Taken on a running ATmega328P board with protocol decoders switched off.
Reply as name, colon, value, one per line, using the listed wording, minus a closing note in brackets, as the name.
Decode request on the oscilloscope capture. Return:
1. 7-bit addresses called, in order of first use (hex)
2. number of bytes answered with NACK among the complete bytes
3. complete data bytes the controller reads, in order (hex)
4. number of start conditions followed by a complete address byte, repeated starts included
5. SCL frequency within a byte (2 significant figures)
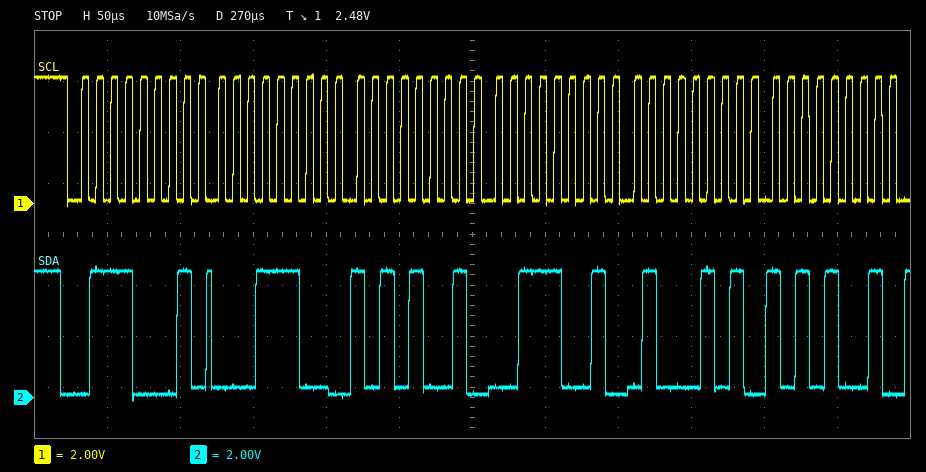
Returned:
7-bit addresses called, in order of first use: 0x38
number of bytes answered with NACK among the complete bytes: 0
complete data bytes the controller reads, in order: 1C A9 39 45 A9
number of start conditions followed by a complete address byte, repeated starts included: 1
SCL frequency within a byte: 100 kHz
